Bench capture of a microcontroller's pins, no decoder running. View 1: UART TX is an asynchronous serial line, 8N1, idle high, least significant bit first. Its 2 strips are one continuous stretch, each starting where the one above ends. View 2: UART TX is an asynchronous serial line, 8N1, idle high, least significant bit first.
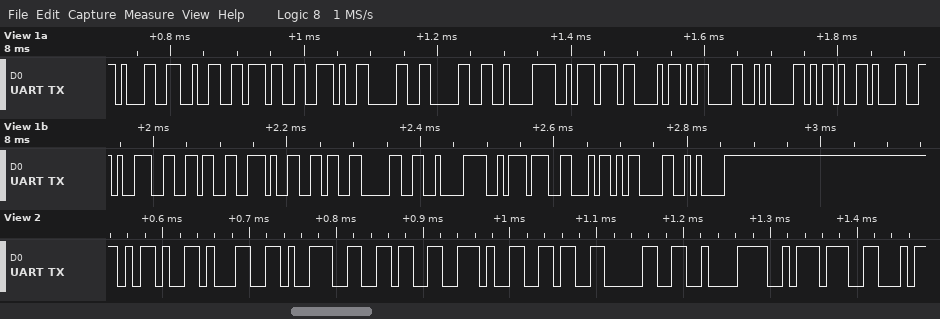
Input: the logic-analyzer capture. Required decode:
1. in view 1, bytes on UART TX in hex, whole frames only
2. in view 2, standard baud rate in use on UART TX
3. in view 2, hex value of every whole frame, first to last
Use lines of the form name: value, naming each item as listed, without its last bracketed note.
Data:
in view 1, bytes on UART TX in hex, whole frames only: 31 32 37 2E 30 30 C2 BA 43 0D 0A 2D 31 39 36 2E 36 30 C2 BA 46 0D 0A
in view 2, standard baud rate in use on UART TX: 115200 baud
in view 2, hex value of every whole frame, first to last: 0x2D 0x31 0x39 0x36 0x2E 0x36 0x30 0xC2 0xBA 0x46
